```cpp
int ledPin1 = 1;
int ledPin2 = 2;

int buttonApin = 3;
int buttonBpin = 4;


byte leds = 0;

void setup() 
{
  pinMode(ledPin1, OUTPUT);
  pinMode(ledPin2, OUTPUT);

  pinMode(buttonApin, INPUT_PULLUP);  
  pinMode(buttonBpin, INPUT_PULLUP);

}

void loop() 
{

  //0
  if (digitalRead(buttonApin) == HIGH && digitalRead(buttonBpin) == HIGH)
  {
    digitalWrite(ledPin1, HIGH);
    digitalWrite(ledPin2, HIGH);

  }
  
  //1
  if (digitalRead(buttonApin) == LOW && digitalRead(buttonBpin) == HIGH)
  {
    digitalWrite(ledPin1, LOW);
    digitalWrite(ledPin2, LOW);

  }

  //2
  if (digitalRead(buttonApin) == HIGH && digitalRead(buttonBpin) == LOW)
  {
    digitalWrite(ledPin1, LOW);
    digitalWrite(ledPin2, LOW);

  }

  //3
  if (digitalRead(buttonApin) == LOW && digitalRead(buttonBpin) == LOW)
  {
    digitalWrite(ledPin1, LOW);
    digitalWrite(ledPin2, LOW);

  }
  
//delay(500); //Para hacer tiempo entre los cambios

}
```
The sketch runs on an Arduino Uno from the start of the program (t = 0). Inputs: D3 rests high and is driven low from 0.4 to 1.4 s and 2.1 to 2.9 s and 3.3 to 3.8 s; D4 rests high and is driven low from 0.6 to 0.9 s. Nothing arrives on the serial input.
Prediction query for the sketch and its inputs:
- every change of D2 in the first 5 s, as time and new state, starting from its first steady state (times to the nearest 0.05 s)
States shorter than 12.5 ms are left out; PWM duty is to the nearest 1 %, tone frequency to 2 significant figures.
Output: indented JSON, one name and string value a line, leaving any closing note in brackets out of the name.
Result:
{
  "every change of D2 in the first 5 s, as time and new state, starting from its first steady state": "0 s high; 0.4 s low; 1.4 s high; 2.1 s low; 2.9 s high; 3.3 s low; 3.8 s high"
}
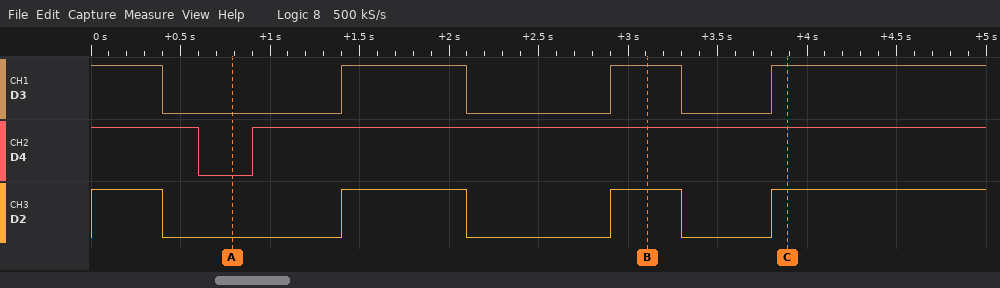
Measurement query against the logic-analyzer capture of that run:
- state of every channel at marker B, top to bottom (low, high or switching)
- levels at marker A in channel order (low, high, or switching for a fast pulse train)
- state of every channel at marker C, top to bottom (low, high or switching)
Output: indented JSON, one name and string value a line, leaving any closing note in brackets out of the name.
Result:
{
  "state of every channel at marker B, top to bottom": "D3 high, D4 high, D2 high",
  "levels at marker A in channel order": "D3 low, D4 low, D2 low",
  "state of every channel at marker C, top to bottom": "D3 high, D4 high, D2 high"
}
